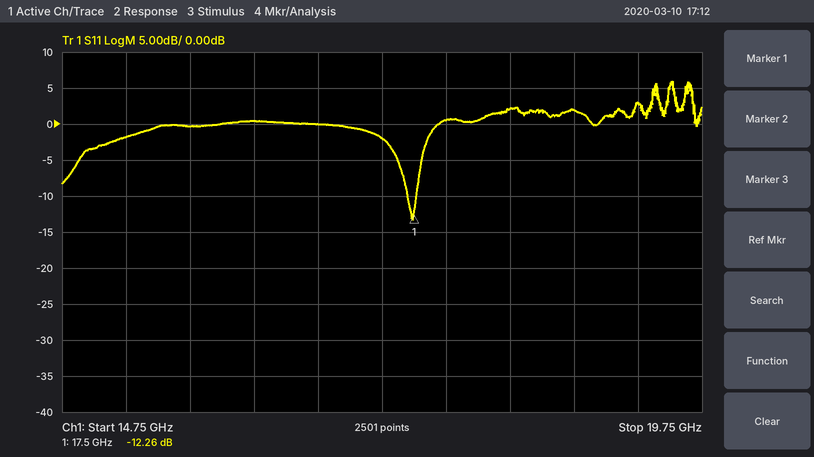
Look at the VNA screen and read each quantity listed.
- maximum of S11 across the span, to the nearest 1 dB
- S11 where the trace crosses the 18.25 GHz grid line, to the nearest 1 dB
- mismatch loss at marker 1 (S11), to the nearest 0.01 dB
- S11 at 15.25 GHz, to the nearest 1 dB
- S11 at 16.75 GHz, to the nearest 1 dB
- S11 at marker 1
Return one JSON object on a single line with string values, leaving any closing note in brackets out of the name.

{"maximum of S11 across the span, to the nearest 1 dB": "6 dB", "S11 where the trace crosses the 18.25 GHz grid line, to the nearest 1 dB": "2 dB", "mismatch loss at marker 1 (S11), to the nearest 0.01 dB": "0.27 dB", "S11 at 15.25 GHz, to the nearest 1 dB": "-2 dB", "S11 at 16.75 GHz, to the nearest 1 dB": "0 dB", "S11 at marker 1": "-12.26 dB"}
